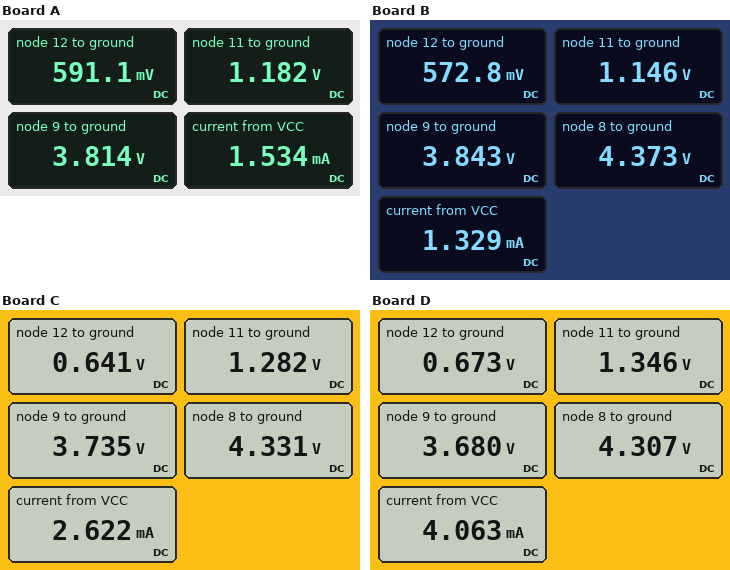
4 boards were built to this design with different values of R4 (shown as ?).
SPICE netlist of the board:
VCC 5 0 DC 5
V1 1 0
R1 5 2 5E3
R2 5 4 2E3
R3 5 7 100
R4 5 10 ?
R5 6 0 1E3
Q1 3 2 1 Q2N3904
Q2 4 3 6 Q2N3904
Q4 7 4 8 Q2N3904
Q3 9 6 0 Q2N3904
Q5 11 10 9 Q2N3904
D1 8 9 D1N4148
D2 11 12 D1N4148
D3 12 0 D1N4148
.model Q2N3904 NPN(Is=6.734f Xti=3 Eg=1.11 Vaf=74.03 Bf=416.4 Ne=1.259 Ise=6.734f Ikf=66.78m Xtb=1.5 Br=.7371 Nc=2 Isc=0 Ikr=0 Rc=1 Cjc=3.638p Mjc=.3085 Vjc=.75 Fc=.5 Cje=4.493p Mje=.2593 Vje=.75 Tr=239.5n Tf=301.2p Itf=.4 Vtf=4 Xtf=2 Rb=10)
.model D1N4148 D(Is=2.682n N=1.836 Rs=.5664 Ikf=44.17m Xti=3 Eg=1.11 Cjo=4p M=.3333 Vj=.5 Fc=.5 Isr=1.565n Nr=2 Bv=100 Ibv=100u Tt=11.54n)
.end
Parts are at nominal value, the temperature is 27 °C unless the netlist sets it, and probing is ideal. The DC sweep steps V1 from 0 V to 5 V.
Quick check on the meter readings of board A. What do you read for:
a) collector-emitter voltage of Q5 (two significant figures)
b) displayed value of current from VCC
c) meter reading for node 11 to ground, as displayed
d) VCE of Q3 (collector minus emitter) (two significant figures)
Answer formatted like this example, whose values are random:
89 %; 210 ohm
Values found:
-2.6 V; 1.534 mA; 1.182 V; 3.8 V
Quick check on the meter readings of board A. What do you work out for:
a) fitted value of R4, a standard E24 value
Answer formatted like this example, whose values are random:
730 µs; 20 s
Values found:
8.2 kΩ
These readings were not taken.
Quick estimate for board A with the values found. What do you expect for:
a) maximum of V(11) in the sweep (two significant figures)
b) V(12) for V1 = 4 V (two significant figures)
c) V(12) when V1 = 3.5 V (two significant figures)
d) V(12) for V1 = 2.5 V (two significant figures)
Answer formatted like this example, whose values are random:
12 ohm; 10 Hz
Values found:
1.2 V; 25 mV; 25 mV; 25 mV
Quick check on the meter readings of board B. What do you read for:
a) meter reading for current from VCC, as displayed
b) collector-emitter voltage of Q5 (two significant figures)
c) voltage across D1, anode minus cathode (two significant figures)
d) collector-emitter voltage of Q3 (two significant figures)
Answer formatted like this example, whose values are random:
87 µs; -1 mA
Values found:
1.329 mA; -2.7 V; 530 mV; 3.8 V
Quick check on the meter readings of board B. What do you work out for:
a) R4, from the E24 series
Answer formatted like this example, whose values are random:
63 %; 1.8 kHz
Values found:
12 kΩ
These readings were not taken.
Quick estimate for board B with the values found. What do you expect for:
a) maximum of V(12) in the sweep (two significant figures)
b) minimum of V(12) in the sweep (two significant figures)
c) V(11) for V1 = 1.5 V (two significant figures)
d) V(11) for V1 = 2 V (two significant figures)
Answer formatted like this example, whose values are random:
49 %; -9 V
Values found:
570 mV; 24 mV; 48 mV; 48 mV
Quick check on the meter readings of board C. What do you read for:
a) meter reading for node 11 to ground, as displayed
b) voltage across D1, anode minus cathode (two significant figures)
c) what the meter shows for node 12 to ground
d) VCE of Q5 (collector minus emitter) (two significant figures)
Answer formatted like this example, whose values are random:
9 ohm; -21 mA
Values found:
1.282 V; 600 mV; 0.641 V; -2.5 V
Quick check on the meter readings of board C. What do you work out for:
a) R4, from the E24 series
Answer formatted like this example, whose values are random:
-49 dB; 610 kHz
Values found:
3 kΩ
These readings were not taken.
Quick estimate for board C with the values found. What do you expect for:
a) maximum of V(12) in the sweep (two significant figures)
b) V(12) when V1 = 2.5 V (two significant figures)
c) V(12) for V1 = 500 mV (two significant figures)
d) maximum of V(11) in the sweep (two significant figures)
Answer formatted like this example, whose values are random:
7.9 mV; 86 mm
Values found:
640 mV; 28 mV; 640 mV; 1.3 V
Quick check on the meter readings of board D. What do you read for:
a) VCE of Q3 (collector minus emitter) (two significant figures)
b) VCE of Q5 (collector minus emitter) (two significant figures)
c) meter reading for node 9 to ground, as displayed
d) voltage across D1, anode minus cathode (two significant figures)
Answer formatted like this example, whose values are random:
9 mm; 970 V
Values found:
3.7 V; -2.3 V; 3.680 V; 630 mV
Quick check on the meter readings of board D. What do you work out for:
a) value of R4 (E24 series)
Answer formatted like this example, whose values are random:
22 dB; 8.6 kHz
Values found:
1.6 kΩ
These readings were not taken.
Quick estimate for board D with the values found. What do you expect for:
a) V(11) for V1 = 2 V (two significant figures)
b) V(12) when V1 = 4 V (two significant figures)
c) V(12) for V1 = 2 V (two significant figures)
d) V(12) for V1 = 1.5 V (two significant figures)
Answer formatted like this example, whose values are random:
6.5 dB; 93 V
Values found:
63 mV; 32 mV; 32 mV; 32 mV
